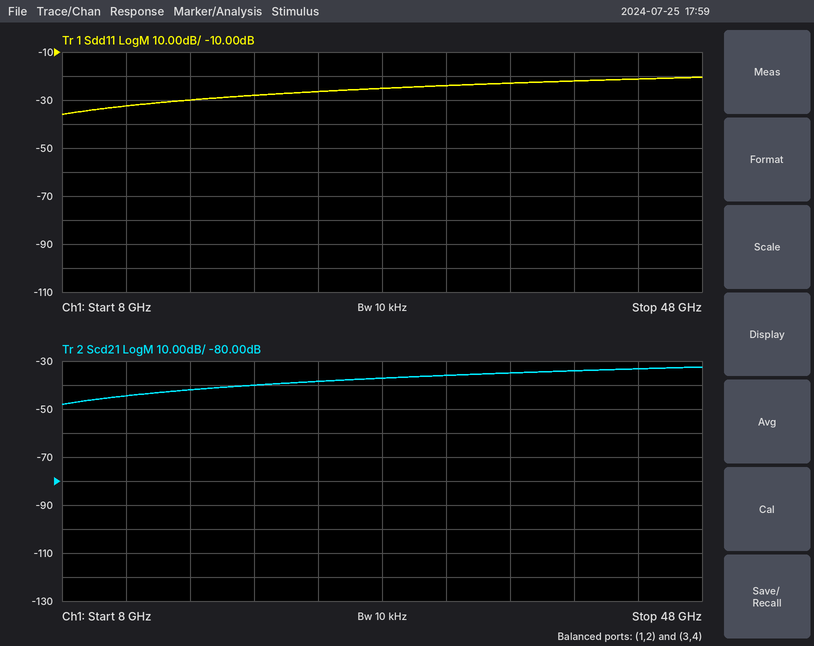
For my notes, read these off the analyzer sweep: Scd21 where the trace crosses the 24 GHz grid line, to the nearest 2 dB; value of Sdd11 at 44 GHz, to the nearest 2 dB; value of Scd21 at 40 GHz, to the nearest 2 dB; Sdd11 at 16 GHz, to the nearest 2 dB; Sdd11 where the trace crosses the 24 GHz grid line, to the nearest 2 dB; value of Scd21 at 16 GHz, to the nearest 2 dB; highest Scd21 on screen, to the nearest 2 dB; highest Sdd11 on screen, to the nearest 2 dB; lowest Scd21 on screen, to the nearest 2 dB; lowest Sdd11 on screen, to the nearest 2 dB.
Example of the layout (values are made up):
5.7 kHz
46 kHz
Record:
-38 dB
-22 dB
-34 dB
-30 dB
-26 dB
-42 dB
-32 dB
-20 dB
-48 dB
-36 dB
